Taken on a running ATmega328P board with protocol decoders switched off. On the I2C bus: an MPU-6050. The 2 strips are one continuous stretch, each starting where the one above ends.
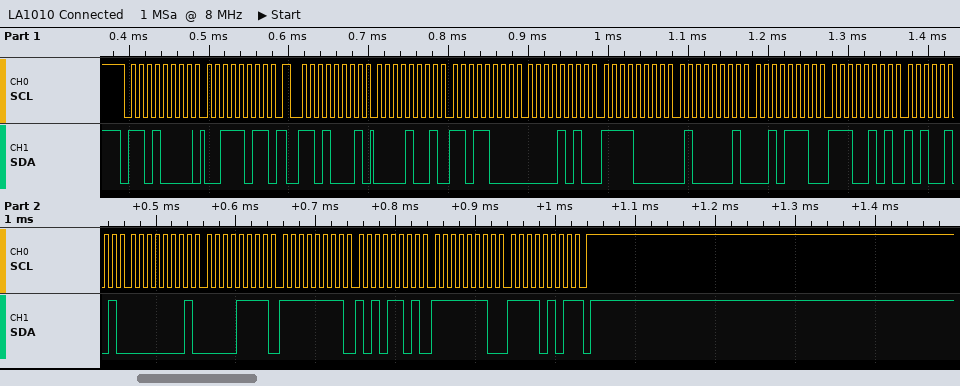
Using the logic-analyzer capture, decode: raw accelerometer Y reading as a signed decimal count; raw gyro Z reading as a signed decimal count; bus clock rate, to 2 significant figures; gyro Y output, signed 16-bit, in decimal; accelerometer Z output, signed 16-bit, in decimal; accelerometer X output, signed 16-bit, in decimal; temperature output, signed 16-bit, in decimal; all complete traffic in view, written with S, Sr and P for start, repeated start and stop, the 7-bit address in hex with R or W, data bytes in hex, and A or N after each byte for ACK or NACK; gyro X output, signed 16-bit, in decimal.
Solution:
2800
-267
100 kHz
-83
16686
2520
-6747
S 68W A 3B A Sr 68R A 09 A D8 A 0A A F0 A 41 A 2E A E5 A A5 A 01 A 0F A FF A AD A FE A F5 N P
271
